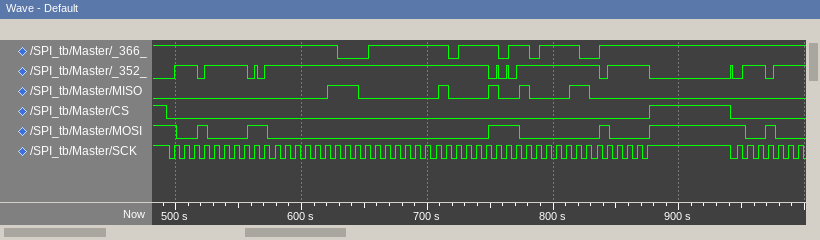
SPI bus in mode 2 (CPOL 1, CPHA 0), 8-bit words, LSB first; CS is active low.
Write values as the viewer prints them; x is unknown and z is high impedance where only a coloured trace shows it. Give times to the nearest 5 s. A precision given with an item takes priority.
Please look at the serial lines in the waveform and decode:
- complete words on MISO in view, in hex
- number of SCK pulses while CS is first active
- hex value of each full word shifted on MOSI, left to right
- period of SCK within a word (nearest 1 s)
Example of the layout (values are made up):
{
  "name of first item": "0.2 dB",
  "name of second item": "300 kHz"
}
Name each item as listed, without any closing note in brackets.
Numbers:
{
  "complete words on MISO in view, in hex": "00, 00, 07, 08, 09, 03",
  "number of SCK pulses while CS is first active": "48",
  "hex value of each full word shifted on MOSI, left to right": "09, 03, 00, 00, 07, 08",
  "period of SCK within a word": "8 s"
}
